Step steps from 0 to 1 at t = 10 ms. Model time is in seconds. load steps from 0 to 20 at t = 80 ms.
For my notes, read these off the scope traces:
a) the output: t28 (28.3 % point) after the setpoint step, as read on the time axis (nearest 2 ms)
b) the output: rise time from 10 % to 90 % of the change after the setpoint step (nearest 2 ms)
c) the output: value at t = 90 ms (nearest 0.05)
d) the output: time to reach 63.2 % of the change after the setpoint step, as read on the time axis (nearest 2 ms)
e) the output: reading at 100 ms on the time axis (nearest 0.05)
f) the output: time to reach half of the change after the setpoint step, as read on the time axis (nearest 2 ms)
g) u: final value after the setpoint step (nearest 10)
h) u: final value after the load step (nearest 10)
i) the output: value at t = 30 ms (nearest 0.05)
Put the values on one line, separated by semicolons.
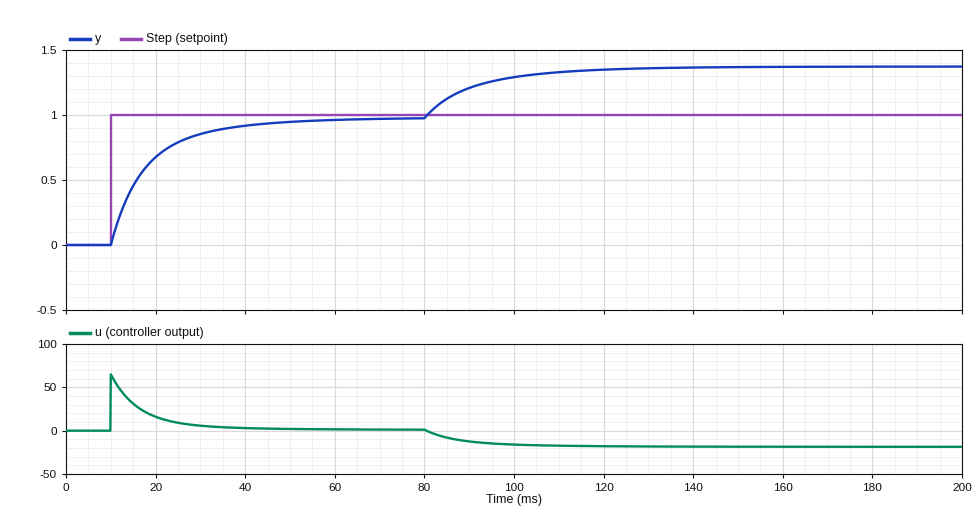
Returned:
12 ms; 22 ms; 1.20; 18 ms; 1.30; 16 ms; 0; -20; 0.85
